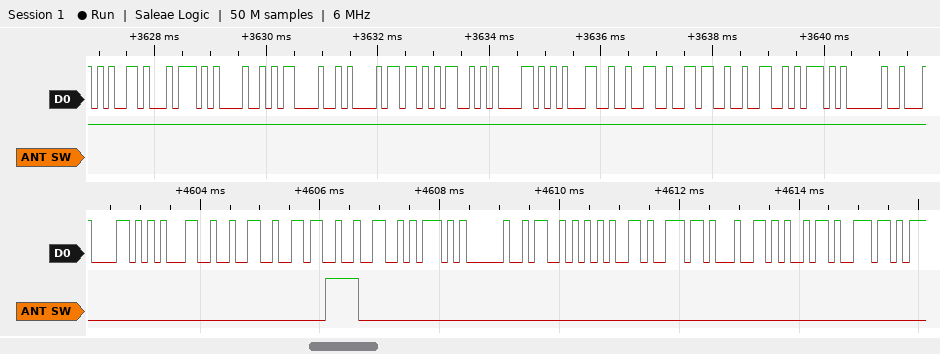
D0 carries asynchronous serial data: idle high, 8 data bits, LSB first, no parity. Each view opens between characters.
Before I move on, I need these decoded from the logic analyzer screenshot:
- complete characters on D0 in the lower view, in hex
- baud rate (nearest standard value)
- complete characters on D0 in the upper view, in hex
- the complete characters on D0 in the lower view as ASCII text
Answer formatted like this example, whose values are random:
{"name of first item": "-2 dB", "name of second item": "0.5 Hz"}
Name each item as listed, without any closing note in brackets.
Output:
{"complete characters on D0 in the lower view, in hex": "58, 31, 32, 36, 32, 5D, 20, 53, 65, 6E, 64, 69, 6E", "baud rate": "9600 baud", "complete characters on D0 in the upper view, in hex": "65, 74, 21, 0D, 0A, 5B, 53, 58, 31, 32, 36, 32, 5D, 20", "the complete characters on D0 in the lower view as ASCII text": "\"X1262] Sendin\""}
